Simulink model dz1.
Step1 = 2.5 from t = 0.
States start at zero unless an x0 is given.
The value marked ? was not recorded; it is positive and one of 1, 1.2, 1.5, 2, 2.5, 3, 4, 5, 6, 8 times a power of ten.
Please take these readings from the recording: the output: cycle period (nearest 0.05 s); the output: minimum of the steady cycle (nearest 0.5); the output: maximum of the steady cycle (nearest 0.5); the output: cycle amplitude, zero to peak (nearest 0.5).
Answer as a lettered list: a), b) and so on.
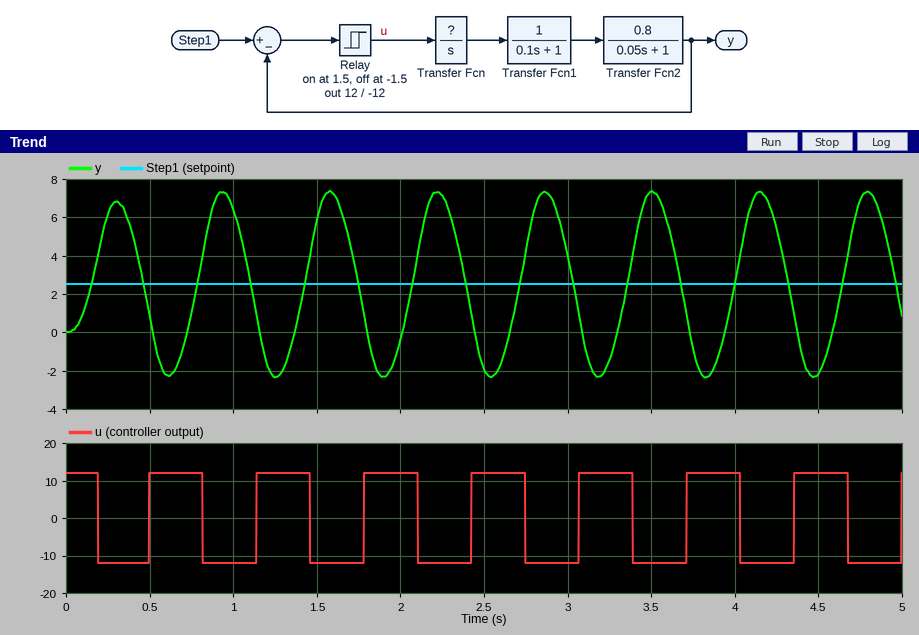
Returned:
a) 0.65 s
b) -2.5
c) 7.5
d) 5.0
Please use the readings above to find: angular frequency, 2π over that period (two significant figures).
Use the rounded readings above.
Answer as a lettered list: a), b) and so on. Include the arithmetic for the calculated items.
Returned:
a) 2π / 0.65 = 9.7 rad/s
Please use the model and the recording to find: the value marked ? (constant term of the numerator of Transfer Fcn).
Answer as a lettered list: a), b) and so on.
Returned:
a) 6
